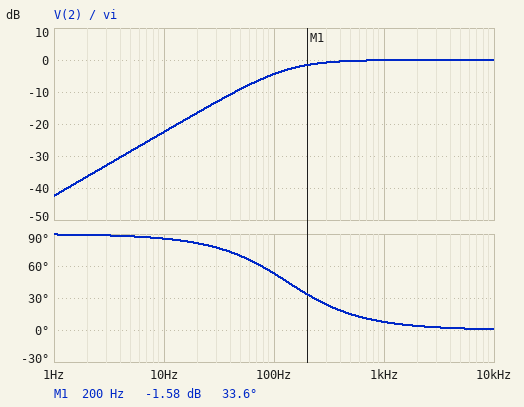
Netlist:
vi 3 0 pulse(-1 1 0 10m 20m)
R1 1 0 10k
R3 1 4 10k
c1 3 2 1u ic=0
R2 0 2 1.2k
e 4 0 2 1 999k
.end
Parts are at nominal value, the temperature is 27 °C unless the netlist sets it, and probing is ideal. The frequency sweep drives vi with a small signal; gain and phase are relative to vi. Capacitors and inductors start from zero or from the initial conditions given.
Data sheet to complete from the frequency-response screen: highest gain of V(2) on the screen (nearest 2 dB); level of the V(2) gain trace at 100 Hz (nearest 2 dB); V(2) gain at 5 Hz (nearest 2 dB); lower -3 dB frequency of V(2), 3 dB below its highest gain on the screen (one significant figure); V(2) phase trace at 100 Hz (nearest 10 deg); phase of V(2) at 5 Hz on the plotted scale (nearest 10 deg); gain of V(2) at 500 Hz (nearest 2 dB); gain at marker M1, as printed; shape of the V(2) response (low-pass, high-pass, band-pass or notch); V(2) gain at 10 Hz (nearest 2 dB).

0 dB
-4 dB
-28 dB
100 Hz
50 deg
90 deg
0 dB
-1.58 dB
high-pass
-22 dB
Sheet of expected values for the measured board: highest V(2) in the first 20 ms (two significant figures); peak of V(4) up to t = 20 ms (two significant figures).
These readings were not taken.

240 mV
480 mV
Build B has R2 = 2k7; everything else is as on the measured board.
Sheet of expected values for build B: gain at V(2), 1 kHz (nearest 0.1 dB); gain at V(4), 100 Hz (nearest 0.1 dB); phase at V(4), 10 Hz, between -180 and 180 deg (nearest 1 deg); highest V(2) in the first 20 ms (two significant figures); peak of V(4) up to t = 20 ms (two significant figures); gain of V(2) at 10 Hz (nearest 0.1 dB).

0 dB
4.7 dB
80 deg
500 mV
1.0 V
-15.5 dB
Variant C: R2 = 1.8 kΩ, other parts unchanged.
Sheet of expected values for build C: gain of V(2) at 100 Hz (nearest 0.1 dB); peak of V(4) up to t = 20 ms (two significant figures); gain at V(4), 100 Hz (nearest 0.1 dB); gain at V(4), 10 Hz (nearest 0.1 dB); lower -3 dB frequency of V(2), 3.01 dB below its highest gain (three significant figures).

-2.5 dB
710 mV
3.5 dB
-13.0 dB
88.4 Hz
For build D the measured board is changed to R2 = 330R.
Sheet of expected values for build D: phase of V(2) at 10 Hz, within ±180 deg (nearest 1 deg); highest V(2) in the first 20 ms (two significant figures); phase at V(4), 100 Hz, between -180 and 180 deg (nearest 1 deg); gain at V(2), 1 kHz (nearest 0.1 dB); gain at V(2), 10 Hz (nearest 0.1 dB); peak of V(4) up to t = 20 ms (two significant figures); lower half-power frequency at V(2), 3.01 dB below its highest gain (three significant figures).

89 deg
66 mV
78 deg
-0.9 dB
-33.7 dB
130 mV
482 Hz
